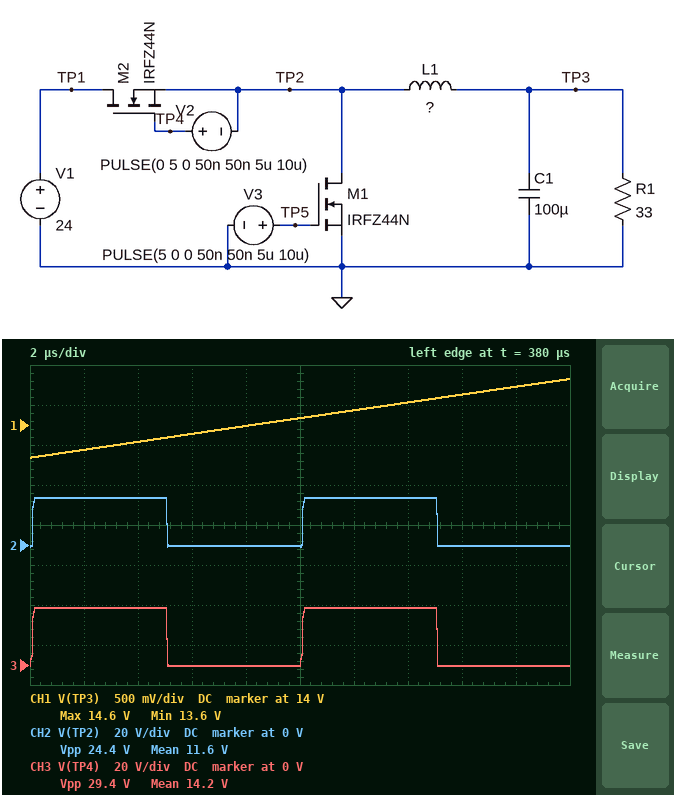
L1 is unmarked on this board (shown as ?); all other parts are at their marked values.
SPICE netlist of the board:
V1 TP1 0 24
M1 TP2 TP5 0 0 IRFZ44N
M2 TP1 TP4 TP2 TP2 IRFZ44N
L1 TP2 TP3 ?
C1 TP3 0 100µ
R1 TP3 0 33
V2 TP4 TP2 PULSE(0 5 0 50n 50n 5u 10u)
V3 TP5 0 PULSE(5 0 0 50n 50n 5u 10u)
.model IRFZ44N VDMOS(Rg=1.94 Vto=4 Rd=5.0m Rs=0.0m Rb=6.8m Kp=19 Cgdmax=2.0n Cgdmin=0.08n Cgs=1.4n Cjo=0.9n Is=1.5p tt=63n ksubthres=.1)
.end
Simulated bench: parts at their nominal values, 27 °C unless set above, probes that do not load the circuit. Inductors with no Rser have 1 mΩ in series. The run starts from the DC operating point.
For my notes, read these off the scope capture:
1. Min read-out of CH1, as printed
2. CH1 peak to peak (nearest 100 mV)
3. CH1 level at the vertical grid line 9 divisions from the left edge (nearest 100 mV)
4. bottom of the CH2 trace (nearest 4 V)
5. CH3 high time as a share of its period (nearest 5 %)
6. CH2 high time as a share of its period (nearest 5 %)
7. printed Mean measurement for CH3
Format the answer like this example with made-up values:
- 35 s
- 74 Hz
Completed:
- 13.6 V
- 1.0 V
- 14.5 V
- 0 V
- 50 %
- 50 %
- 14.2 V
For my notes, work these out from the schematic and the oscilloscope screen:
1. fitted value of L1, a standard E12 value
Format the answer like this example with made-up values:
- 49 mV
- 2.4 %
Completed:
- 470 µH
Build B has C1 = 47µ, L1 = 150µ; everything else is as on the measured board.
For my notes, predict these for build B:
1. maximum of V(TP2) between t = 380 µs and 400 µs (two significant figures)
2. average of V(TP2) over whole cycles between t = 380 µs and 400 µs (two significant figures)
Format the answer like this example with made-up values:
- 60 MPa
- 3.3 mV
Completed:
- 25 V
- 13 V
